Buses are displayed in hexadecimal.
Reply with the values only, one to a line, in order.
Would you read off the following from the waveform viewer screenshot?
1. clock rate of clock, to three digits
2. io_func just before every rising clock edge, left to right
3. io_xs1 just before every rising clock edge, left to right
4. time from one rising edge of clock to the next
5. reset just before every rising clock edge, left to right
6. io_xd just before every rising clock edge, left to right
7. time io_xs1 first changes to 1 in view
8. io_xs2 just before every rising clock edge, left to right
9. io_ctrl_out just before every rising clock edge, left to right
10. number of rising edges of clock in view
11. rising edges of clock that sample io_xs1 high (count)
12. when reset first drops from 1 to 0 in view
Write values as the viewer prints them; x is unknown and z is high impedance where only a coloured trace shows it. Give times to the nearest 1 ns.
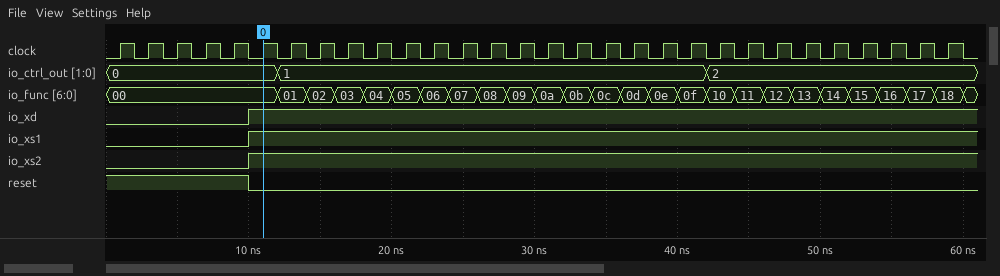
500 MHz
00, 00, 00, 00, 00, 00, 01, 02, 03, 04, 05, 06, 07, 08, 09, 0a, 0b, 0c, 0d, 0e, 0f, 10, 11, 12, 13, 14, 15, 16, 17, 18
0 0 0 0 0 1 1 1 1 1 1 1 1 1 1 1 1 1 1 1 1 1 1 1 1 1 1 1 1 1
2 ns
1 1 1 1 1 0 0 0 0 0 0 0 0 0 0 0 0 0 0 0 0 0 0 0 0 0 0 0 0 0
0 0 0 0 0 1 1 1 1 1 1 1 1 1 1 1 1 1 1 1 1 1 1 1 1 1 1 1 1 1
10 ns
0 0 0 0 0 1 1 1 1 1 1 1 1 1 1 1 1 1 1 1 1 1 1 1 1 1 1 1 1 1
0, 0, 0, 0, 0, 0, 1, 1, 1, 1, 1, 1, 1, 1, 1, 1, 1, 1, 1, 1, 1, 2, 2, 2, 2, 2, 2, 2, 2, 2
30
25
10 ns
